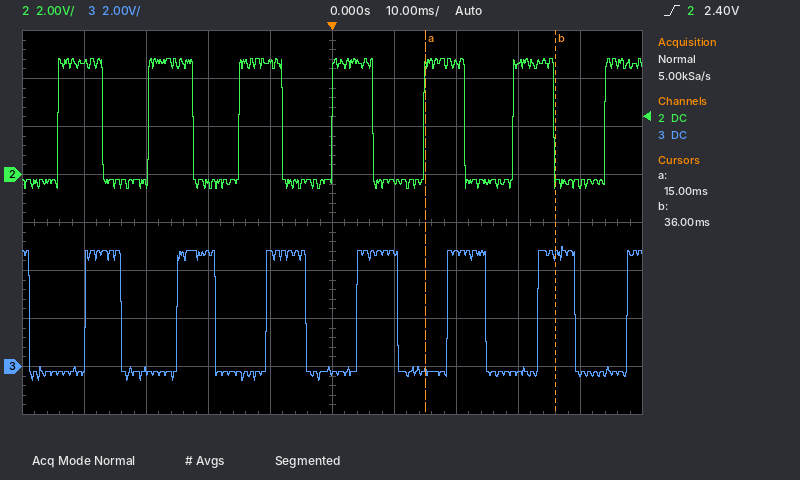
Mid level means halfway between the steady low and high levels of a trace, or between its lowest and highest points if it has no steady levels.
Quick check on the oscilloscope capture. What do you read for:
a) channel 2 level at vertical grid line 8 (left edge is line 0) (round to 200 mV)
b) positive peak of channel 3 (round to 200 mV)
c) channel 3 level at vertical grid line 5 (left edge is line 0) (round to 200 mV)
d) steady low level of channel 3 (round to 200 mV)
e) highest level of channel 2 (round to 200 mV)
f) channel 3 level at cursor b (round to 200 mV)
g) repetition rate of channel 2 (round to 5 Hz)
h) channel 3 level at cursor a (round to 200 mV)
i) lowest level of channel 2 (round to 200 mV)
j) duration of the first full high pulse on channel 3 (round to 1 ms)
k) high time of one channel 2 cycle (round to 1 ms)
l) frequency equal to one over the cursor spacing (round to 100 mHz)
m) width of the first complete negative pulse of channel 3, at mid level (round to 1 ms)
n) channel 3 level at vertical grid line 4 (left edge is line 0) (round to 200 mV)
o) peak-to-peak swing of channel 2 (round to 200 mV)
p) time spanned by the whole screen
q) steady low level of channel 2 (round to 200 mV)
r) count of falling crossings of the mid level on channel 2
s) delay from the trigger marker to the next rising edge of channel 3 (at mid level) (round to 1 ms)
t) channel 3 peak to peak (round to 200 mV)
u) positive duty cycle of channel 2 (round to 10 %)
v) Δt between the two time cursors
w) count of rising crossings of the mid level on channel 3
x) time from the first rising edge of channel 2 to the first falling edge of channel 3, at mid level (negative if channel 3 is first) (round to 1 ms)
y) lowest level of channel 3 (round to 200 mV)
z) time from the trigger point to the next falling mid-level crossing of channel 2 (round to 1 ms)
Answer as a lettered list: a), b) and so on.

a) 4.6 V
b) 5.0 V
c) -200 mV
d) -200 mV
e) 4.8 V
f) 4.6 V
g) 70 Hz
h) -200 mV
i) -600 mV
j) 6 ms
k) 7 ms
l) 47.6 Hz
m) 9 ms
n) 4.8 V
o) 5.4 V
p) 100 ms
q) -200 mV
r) 6
s) 4 ms
t) 5.6 V
u) 50 %
v) 21 ms
w) 7
x) -5 ms
y) -600 mV
z) 7 ms
